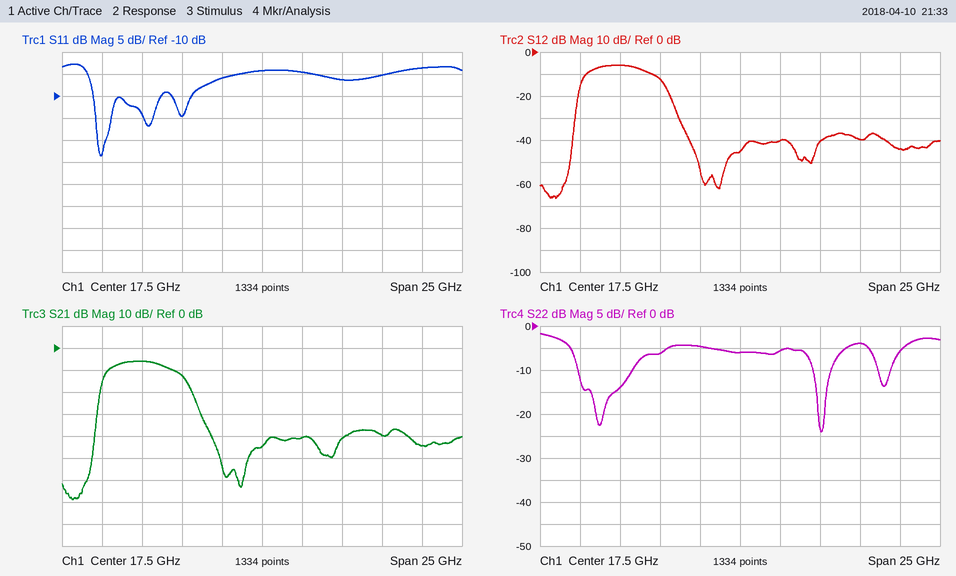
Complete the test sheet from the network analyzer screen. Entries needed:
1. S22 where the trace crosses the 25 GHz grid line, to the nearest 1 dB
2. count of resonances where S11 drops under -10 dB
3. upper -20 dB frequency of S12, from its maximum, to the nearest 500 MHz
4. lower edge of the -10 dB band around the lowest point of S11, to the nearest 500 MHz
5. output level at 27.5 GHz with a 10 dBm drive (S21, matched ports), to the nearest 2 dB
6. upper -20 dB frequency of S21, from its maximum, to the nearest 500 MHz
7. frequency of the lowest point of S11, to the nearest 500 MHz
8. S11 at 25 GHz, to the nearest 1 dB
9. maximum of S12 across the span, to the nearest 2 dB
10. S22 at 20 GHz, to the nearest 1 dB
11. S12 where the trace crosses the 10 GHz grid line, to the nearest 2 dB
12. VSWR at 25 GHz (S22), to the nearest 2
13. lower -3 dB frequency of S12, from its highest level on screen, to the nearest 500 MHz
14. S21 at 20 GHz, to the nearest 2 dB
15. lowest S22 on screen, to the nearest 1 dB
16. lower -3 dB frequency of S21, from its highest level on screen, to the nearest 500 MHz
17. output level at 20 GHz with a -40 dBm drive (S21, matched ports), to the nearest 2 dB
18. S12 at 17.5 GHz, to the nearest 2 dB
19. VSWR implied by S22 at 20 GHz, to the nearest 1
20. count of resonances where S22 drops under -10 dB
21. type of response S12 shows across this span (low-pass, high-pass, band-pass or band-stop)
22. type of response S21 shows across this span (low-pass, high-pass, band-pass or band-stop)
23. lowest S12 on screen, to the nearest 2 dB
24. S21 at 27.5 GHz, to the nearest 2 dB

-4 dB
3
13.5 GHz
7.0 GHz
-34 dBm
13.5 GHz
7.5 GHz
-5 dB
-6 dB
-6 dB
-6 dB
4
8.0 GHz
-40 dB
-24 dB
8.0 GHz
-80 dBm
-46 dB
3
3
band-pass
band-pass
-66 dB
-44 dB
